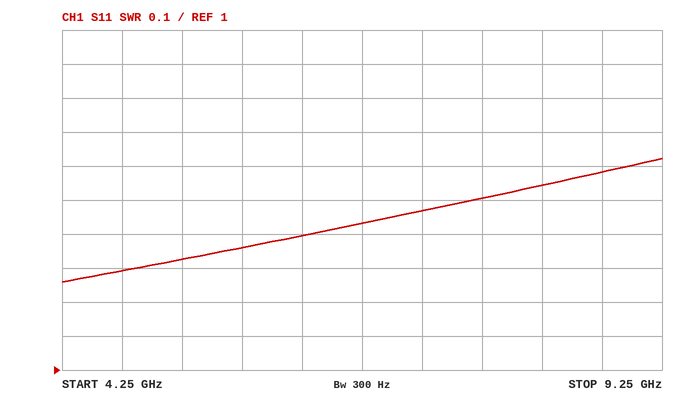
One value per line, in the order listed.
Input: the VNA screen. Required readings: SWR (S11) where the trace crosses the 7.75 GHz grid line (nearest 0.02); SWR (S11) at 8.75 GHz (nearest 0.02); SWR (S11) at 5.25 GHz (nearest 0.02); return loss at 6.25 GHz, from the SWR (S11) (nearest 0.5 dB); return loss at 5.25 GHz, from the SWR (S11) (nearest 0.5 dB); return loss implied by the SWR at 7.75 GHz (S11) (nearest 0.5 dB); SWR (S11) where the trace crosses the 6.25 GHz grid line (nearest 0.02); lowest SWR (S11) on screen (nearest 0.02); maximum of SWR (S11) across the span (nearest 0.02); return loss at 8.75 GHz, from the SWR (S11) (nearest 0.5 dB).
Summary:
1.50
1.58
1.32
15.5 dB
17.0 dB
14.0 dB
1.40
1.26
1.62
13.0 dB
